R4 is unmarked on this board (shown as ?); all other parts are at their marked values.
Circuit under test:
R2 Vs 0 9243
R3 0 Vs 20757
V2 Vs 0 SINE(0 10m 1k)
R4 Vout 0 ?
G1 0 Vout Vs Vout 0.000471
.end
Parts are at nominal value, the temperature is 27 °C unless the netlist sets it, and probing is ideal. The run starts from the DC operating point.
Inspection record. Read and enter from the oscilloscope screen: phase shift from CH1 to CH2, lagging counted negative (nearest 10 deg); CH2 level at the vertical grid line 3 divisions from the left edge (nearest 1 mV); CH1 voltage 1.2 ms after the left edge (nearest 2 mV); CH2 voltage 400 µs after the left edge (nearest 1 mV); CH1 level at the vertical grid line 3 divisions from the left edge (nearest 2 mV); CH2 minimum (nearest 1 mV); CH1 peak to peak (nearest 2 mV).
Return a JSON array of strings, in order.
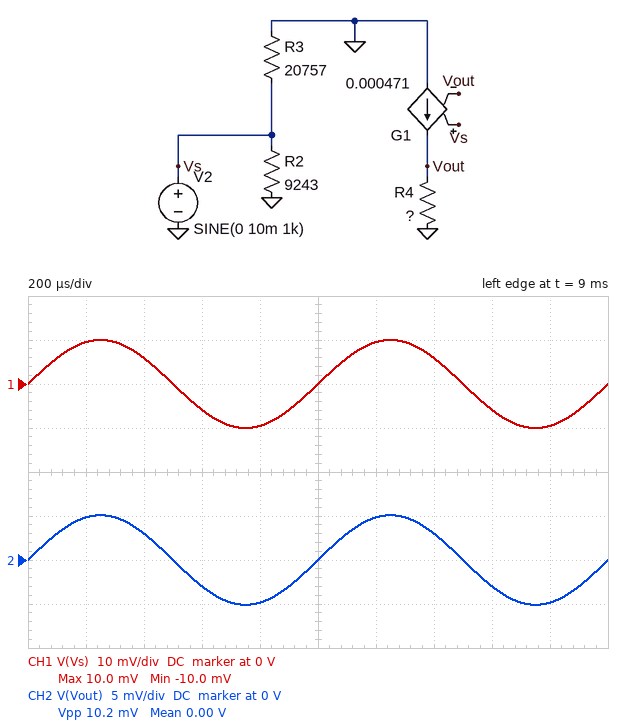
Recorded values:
["0 deg", "-3 mV", "10 mV", "3 mV", "-6 mV", "-5 mV", "20 mV"]
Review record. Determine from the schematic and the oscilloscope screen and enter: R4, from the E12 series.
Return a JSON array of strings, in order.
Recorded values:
["2.2 kΩ"]
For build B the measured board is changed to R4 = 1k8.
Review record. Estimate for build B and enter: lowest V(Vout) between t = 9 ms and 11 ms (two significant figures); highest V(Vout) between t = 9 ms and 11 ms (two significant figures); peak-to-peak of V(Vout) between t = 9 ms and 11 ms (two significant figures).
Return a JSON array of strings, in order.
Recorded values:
["-4.6 mV", "4.6 mV", "9.2 mV"]
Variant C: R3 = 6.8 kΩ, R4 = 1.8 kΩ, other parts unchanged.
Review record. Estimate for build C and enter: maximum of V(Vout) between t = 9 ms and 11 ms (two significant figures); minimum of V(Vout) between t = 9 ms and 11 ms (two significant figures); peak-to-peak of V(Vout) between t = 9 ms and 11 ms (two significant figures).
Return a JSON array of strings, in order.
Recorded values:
["4.6 mV", "-4.6 mV", "9.2 mV"]
